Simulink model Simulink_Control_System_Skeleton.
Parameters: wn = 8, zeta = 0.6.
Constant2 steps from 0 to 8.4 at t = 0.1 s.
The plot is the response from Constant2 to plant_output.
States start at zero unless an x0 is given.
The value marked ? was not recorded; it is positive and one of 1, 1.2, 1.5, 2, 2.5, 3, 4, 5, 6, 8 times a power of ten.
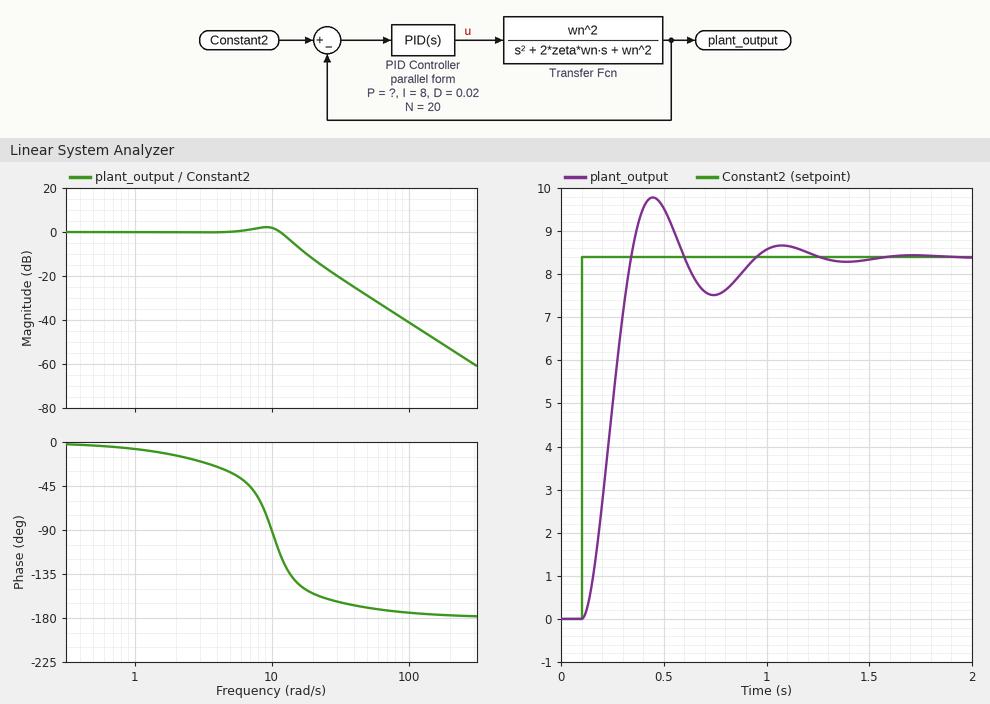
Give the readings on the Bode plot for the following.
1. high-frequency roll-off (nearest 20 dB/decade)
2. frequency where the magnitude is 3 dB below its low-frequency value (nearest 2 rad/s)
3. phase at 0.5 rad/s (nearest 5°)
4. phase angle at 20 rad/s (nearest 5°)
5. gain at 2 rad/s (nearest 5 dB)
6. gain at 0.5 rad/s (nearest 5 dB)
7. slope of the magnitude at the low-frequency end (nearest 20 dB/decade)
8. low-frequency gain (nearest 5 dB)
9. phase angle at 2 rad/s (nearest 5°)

-40 dB/decade
14 rad/s
-5°
-155°
0 dB
0 dB
0 dB/decade
0 dB
-15°
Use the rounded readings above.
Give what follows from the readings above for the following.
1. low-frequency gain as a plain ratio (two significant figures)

1.0
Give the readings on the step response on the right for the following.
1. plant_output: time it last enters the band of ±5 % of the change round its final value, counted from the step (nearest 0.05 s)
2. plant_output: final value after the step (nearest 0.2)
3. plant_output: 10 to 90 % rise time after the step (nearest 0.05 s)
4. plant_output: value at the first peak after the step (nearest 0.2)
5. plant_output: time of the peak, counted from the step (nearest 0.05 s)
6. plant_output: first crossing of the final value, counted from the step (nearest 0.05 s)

0.75 s
8.4
0.15 s
9.8
0.35 s
0.25 s
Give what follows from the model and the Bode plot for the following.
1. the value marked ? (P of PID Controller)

1
